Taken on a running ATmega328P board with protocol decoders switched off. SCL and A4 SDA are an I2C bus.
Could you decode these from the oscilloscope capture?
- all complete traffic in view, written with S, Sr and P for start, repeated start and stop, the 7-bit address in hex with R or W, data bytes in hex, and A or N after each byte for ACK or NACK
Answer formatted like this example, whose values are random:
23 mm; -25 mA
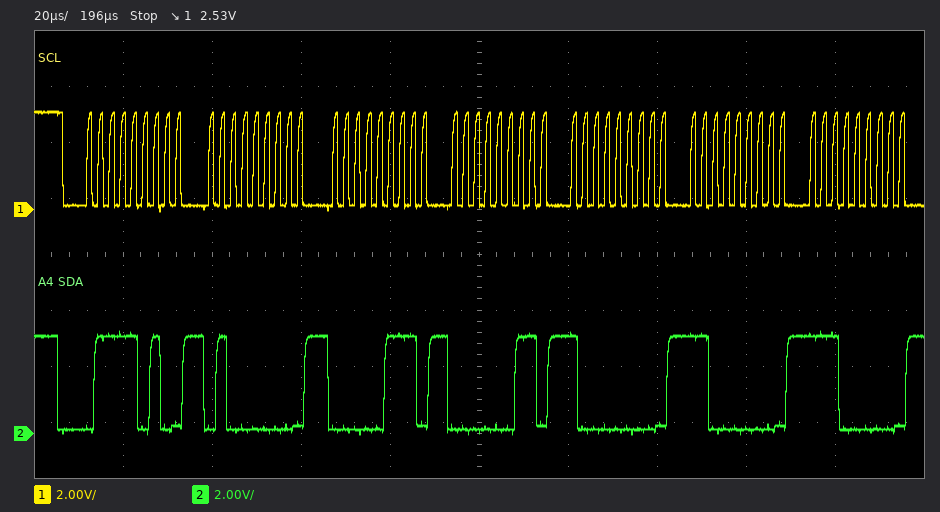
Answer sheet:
S 3DW A 40 A 07 A 03 A 80 A C0 A E0 A
